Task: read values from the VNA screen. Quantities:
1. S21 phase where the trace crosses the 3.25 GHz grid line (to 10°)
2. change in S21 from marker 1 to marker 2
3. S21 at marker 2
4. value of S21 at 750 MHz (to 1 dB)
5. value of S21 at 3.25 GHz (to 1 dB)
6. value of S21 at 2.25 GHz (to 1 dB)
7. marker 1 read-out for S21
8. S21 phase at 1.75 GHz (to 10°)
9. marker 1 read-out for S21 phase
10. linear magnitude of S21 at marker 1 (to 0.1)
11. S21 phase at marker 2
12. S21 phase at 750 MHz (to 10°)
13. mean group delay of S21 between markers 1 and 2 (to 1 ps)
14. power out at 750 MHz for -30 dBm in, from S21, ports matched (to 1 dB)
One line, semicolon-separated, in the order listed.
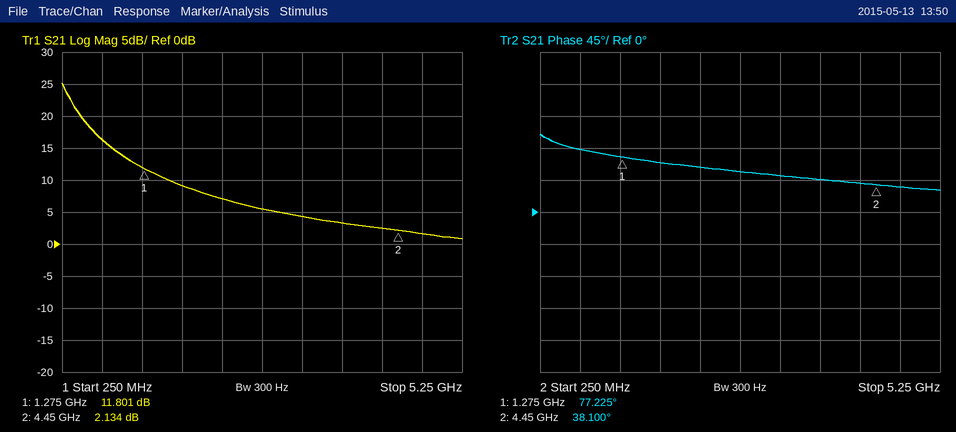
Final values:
50°; -9.667 dB; 2.134 dB; 16 dB; 4 dB; 7 dB; 11.801 dB; 70°; 77.225°; 3.9; 38.100°; 90°; 34 ps; -14 dBm
